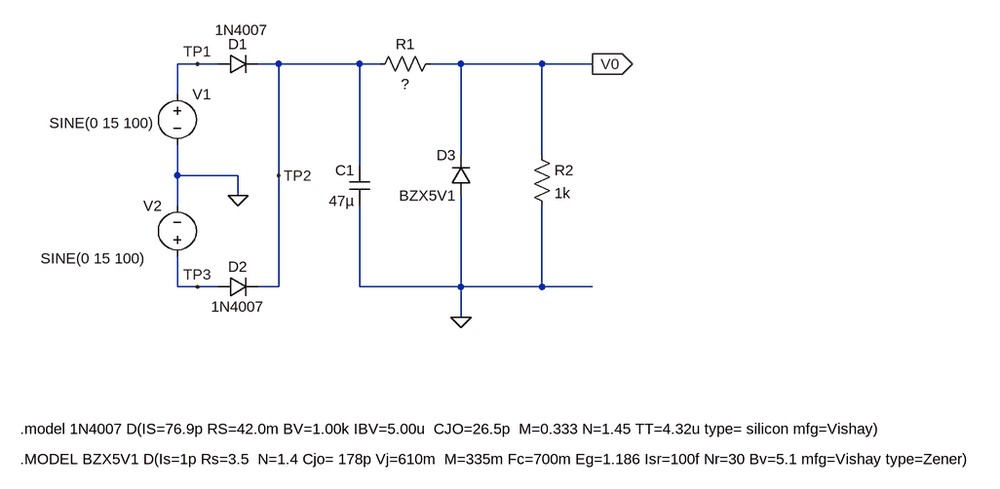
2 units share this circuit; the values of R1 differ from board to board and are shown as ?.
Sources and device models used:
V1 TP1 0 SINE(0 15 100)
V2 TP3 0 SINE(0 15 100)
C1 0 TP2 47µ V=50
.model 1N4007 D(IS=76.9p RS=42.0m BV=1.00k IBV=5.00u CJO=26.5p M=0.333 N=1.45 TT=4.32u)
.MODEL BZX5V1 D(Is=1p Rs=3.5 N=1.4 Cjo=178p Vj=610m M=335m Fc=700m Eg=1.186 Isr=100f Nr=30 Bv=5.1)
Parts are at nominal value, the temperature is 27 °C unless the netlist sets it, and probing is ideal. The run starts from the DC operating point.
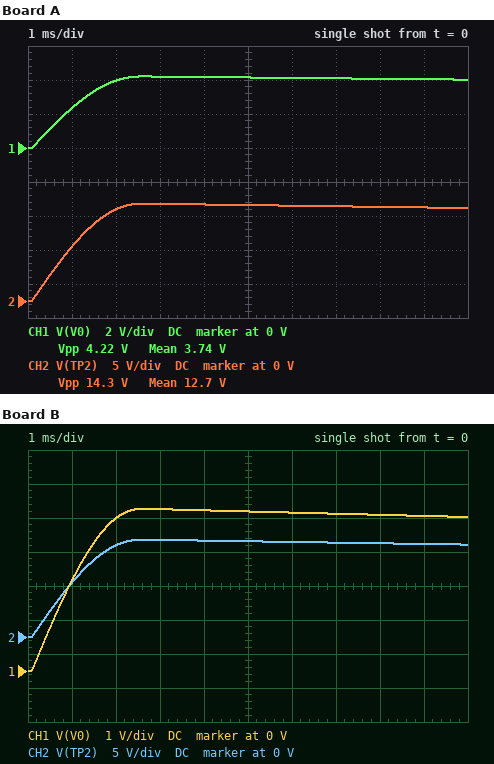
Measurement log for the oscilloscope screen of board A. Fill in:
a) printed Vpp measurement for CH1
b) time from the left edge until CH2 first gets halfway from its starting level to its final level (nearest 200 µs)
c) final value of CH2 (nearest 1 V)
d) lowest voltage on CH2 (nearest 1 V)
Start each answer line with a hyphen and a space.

- 4.22 V
- 800 µs
- 14 V
- 0 V
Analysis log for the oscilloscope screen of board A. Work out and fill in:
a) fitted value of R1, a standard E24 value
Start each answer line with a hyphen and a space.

- 2.4 kΩ
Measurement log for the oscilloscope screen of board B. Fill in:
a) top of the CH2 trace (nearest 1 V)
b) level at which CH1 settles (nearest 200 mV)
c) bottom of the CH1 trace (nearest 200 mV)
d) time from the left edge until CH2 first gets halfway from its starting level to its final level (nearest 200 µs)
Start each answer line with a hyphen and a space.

- 14 V
- 4.6 V
- 0 V
- 800 µs
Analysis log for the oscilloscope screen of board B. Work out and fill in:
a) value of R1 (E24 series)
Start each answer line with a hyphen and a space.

- 2 kΩ
